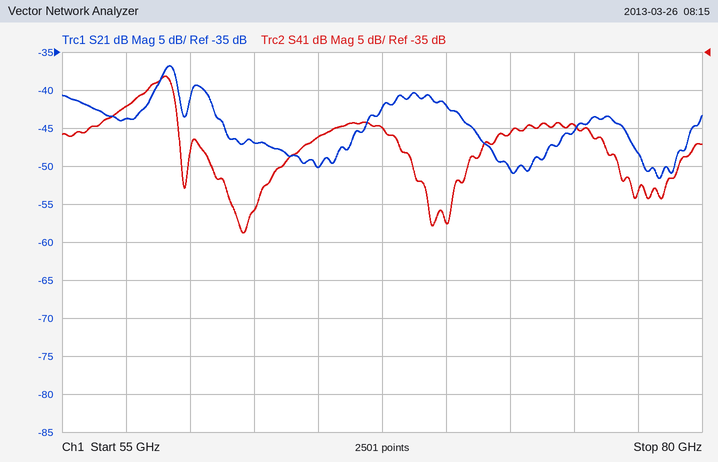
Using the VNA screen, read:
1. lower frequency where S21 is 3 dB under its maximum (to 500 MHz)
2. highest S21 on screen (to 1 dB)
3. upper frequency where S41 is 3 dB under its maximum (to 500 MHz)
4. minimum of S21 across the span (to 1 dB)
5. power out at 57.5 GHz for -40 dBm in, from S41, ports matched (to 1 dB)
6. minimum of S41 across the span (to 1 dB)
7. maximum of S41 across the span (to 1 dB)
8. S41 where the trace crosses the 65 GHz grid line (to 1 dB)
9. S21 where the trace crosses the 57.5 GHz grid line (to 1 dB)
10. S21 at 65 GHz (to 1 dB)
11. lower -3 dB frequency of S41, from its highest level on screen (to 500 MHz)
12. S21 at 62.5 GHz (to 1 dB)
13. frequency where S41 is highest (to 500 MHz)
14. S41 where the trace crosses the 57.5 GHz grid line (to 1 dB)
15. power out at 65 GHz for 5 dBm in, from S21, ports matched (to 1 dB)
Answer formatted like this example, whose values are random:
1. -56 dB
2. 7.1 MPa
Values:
1. 58.5 GHz
2. -37 dB
3. 59.5 GHz
4. -52 dB
5. -82 dBm
6. -59 dB
7. -38 dB
8. -46 dB
9. -44 dB
10. -50 dB
11. 58.0 GHz
12. -47 dB
13. 59.0 GHz
14. -42 dB
15. -45 dBm
